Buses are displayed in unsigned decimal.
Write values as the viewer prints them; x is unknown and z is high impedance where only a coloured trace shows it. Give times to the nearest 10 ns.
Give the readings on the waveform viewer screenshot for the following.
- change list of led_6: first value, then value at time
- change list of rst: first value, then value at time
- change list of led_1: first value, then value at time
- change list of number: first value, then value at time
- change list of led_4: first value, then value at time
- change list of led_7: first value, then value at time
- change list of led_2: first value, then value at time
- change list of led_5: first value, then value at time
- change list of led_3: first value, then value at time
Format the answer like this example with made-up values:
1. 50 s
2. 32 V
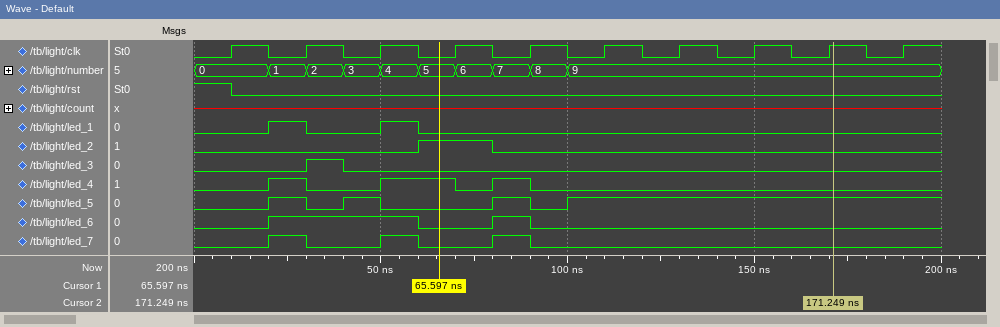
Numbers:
1. 0, 1 at 20 ns, 0 at 60 ns, 1 at 80 ns, 0 at 90 ns
2. 1, 0 at 10 ns
3. 0, 1 at 20 ns, 0 at 30 ns, 1 at 50 ns, 0 at 60 ns
4. 0, 1 at 20 ns, 2 at 30 ns, 3 at 40 ns, 4 at 50 ns, 5 at 60 ns, 6 at 70 ns, 7 at 80 ns, 8 at 90 ns, 9 at 100 ns
5. 0, 1 at 20 ns, 0 at 30 ns, 1 at 50 ns, 0 at 70 ns, 1 at 80 ns, 0 at 90 ns
6. 0, 1 at 20 ns, 0 at 30 ns, 1 at 50 ns, 0 at 60 ns, 1 at 80 ns, 0 at 90 ns
7. 0, 1 at 60 ns, 0 at 80 ns
8. 0, 1 at 20 ns, 0 at 30 ns, 1 at 40 ns, 0 at 50 ns, 1 at 80 ns, 0 at 90 ns, 1 at 100 ns
9. 0, 1 at 30 ns, 0 at 40 ns
